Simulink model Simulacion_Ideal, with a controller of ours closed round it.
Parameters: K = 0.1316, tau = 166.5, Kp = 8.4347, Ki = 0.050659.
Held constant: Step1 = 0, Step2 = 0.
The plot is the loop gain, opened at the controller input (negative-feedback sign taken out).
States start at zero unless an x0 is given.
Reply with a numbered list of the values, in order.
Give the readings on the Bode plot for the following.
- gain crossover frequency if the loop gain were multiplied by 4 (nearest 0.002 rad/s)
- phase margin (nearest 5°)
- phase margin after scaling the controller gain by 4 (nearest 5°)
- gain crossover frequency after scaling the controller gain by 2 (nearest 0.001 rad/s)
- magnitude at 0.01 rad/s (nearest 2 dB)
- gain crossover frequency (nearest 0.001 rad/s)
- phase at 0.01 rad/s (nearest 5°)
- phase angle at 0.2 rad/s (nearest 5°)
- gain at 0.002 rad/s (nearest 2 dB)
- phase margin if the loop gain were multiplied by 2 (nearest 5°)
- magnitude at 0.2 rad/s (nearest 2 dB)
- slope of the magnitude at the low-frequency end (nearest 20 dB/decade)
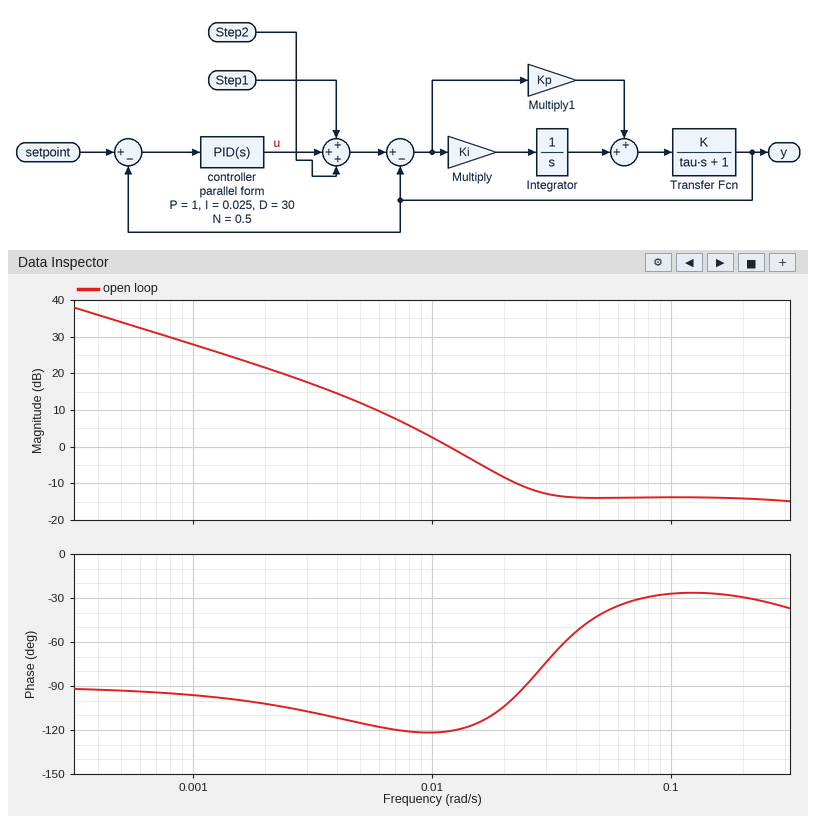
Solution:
1. 0.028 rad/s
2. 60°
3. 100°
4. 0.017 rad/s
5. 2 dB
6. 0.012 rad/s
7. -120°
8. -30°
9. 22 dB
10. 70°
11. -14 dB
12. -20 dB/decade
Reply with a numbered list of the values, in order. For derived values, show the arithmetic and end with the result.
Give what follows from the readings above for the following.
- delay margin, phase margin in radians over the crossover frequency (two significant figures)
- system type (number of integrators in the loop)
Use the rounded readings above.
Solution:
1. 60 × π / 180 / 0.012 = 87 s
2. 1
